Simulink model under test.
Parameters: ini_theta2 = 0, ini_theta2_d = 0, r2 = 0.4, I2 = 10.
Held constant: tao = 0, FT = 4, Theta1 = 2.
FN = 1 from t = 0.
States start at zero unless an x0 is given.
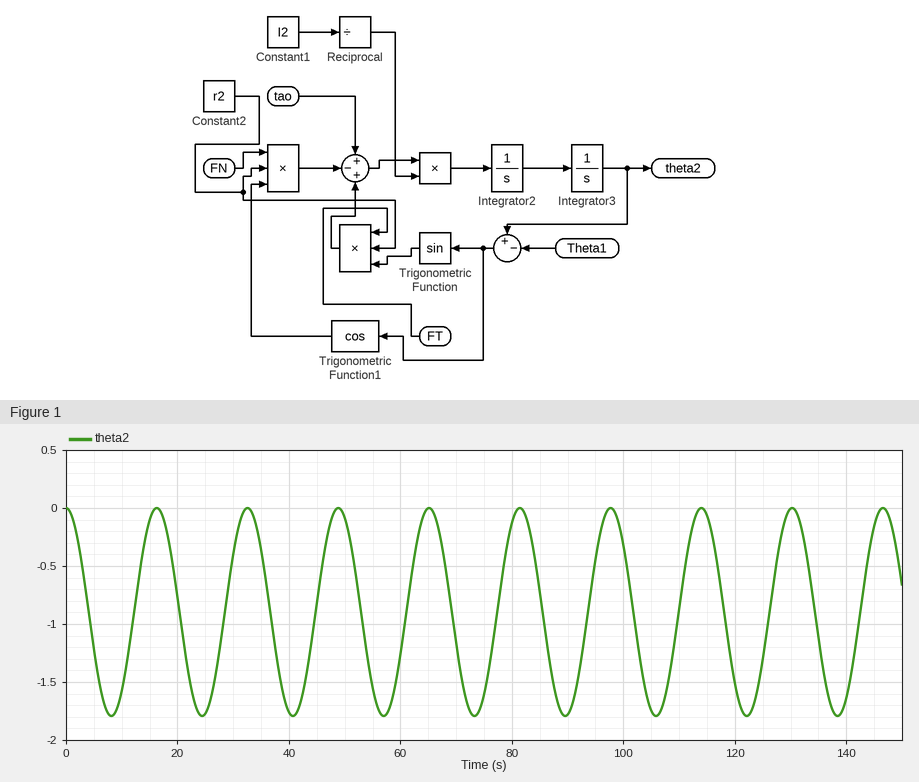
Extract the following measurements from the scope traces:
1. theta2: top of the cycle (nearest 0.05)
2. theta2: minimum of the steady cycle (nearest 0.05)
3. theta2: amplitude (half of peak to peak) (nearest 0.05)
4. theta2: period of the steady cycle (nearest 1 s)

0.00
-1.80
0.90
16 s
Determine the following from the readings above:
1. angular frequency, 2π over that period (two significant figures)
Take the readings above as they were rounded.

0.39 rad/s
